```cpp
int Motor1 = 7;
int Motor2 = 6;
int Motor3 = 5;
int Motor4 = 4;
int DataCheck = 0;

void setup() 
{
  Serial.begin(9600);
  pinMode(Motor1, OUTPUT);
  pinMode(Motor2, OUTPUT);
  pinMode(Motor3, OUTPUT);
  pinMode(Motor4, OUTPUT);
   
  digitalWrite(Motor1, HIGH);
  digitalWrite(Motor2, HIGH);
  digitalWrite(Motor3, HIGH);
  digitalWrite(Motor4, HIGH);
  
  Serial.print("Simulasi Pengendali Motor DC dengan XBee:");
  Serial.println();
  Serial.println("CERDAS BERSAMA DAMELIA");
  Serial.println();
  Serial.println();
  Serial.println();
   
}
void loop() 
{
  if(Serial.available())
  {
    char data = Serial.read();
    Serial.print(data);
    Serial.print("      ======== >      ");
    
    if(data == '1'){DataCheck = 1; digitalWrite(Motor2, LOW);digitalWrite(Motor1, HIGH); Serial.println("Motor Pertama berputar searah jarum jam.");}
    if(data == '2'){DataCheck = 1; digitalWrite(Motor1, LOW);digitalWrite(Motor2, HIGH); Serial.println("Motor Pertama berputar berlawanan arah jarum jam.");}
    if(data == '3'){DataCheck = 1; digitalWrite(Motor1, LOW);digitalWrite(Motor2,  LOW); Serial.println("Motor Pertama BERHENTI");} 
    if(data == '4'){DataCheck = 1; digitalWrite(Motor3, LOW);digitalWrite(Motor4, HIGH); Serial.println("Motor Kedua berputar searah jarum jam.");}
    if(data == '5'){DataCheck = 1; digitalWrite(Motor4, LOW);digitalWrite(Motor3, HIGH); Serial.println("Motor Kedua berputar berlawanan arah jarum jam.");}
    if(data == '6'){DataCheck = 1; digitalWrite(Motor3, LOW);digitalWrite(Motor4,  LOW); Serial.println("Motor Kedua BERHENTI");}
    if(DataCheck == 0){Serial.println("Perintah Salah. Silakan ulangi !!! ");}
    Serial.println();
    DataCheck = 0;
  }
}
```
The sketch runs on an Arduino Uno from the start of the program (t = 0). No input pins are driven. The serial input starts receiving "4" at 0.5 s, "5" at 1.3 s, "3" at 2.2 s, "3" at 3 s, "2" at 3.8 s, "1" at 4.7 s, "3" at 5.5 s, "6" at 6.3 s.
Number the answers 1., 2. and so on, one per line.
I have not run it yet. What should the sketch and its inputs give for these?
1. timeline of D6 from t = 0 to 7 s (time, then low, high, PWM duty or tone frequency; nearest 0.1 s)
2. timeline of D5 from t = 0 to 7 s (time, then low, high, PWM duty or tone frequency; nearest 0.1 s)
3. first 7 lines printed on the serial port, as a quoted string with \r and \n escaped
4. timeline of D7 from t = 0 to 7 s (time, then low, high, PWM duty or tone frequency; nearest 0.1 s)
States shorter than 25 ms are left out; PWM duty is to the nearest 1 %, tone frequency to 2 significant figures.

1. 0 s high; 2.2 s low; 3.8 s high; 4.7 s low
2. 0 s high; 0.5 s low; 1.3 s high; 6.3 s low
3. "Simulasi Pengendali Motor DC dengan XBee:\r\nCERDAS BERSAMA DAMELIA\r\n\r\n\r\n\r\n4      ======== >      Motor Kedua berputar searah jarum jam.\r\n\r\n"
4. 0 s high; 2.2 s low; 4.7 s high; 5.5 s low
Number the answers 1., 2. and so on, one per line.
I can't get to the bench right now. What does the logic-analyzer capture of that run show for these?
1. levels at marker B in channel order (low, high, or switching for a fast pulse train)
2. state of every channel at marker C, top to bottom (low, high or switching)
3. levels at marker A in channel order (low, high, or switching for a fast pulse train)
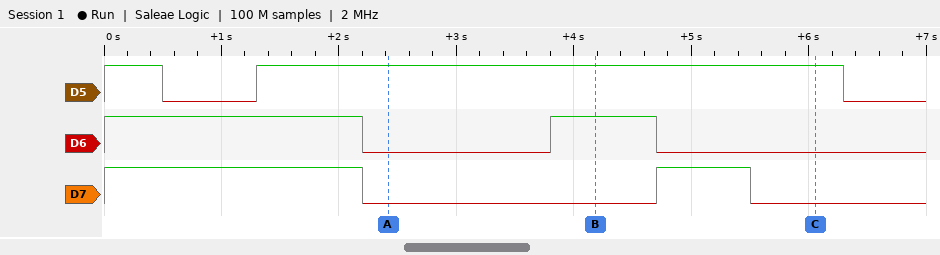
1. D5 high, D6 high, D7 low
2. D5 high, D6 low, D7 low
3. D5 high, D6 low, D7 low
